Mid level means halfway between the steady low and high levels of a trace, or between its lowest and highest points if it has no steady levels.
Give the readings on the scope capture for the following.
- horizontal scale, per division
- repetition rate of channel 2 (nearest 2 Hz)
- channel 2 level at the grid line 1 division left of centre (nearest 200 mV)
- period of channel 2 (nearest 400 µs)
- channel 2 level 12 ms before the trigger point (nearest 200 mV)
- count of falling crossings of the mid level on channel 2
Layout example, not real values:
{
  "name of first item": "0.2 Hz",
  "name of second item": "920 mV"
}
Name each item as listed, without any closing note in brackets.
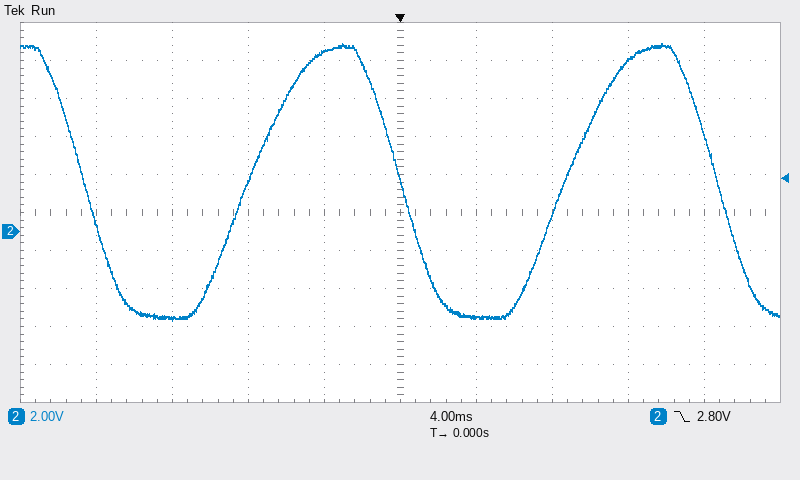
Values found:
{
  "horizontal scale, per division": "4 ms",
  "repetition rate of channel 2": "60 Hz",
  "channel 2 level at the grid line 1 division left of centre": "9.4 V",
  "period of channel 2": "16.8 ms",
  "channel 2 level 12 ms before the trigger point": "-4.6 V",
  "count of falling crossings of the mid level on channel 2": "3"
}
